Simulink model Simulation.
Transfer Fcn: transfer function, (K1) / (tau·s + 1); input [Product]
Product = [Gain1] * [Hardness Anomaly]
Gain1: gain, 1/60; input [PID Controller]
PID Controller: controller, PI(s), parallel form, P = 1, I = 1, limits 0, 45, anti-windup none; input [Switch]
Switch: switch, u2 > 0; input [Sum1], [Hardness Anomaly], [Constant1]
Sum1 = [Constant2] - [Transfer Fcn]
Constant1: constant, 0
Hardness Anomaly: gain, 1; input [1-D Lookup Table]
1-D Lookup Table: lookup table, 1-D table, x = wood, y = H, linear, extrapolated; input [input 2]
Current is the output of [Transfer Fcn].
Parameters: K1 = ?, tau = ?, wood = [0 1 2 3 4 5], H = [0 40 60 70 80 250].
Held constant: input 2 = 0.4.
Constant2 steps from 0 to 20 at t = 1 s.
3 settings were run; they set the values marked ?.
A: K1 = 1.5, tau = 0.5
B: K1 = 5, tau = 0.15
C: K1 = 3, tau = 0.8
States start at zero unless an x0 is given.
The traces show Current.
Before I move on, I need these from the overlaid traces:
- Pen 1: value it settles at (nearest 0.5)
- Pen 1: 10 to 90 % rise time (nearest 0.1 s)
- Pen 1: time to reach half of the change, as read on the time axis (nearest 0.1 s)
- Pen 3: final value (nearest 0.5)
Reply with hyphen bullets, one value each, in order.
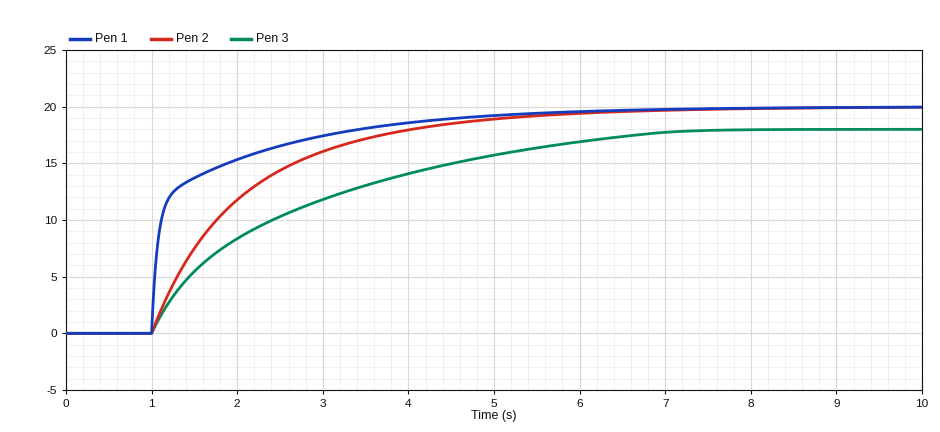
- 20.0
- 2.4 s
- 1.1 s
- 18.0
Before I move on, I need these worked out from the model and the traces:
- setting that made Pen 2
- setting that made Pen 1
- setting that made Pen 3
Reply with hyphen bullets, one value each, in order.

- C
- B
- A
